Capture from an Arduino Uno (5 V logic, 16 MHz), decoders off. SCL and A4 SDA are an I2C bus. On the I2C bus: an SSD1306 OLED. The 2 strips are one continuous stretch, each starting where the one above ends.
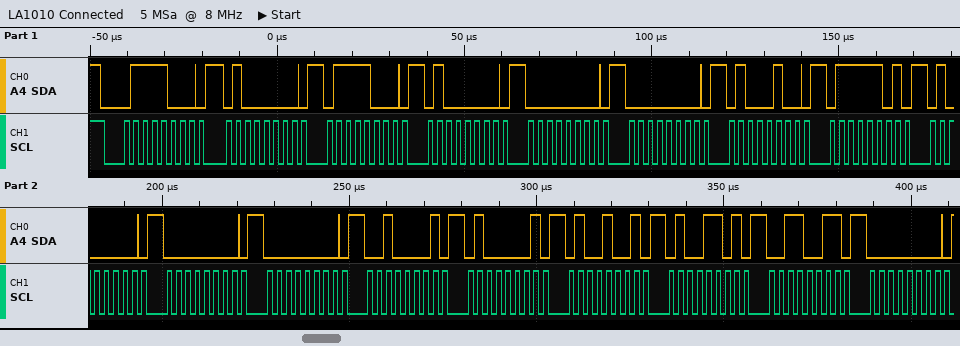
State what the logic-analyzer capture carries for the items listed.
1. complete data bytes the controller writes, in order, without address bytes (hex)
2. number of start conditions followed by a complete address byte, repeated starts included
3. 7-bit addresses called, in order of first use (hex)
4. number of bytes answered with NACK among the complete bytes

40 78 40 00 00 44 7D 40 00 00 21 41 49 4D 33 00
1
0x3C
0
